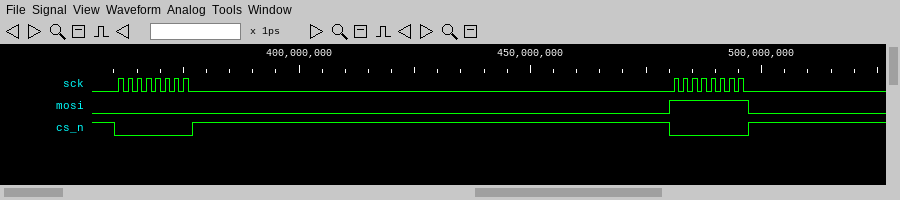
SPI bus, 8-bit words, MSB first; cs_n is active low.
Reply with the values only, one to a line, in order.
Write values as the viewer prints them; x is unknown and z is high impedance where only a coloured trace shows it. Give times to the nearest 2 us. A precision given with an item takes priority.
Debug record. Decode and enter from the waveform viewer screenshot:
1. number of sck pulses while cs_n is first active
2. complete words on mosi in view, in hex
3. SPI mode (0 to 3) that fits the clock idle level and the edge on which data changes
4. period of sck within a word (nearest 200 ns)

8
00, FF
0
2000 ns
